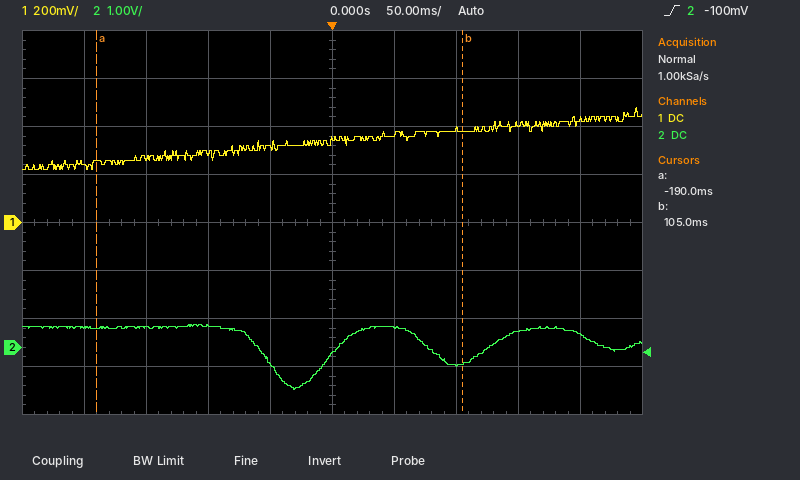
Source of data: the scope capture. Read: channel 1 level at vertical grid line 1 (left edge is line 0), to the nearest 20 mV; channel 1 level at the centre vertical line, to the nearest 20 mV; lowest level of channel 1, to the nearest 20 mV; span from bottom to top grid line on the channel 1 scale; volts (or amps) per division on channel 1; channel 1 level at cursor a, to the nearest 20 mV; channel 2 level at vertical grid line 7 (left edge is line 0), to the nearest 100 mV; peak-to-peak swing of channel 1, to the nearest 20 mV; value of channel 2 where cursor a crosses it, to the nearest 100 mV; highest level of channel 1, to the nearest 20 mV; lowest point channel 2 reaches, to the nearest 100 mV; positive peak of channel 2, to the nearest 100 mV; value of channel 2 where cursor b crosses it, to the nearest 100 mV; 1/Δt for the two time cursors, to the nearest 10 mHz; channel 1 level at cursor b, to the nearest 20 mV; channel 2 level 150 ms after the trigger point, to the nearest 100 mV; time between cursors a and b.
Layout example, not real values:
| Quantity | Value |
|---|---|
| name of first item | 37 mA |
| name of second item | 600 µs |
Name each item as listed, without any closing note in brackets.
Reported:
| Quantity | Value |
|---|---|
| channel 1 level at vertical grid line 1 (left edge is line 0), to the nearest 20 mV | 240 mV |
| channel 1 level at the centre vertical line, to the nearest 20 mV | 340 mV |
| lowest level of channel 1, to the nearest 20 mV | 220 mV |
| span from bottom to top grid line on the channel 1 scale | 1.6 V |
| volts (or amps) per division on channel 1 | 200 mV |
| channel 1 level at cursor a, to the nearest 20 mV | 260 mV |
| channel 2 level at vertical grid line 7 (left edge is line 0), to the nearest 100 mV | -400 mV |
| peak-to-peak swing of channel 1, to the nearest 20 mV | 260 mV |
| value of channel 2 where cursor a crosses it, to the nearest 100 mV | 400 mV |
| highest level of channel 1, to the nearest 20 mV | 480 mV |
| lowest point channel 2 reaches, to the nearest 100 mV | -900 mV |
| positive peak of channel 2, to the nearest 100 mV | 500 mV |
| value of channel 2 where cursor b crosses it, to the nearest 100 mV | -300 mV |
| 1/Δt for the two time cursors, to the nearest 10 mHz | 3.39 Hz |
| channel 1 level at cursor b, to the nearest 20 mV | 380 mV |
| channel 2 level 150 ms after the trigger point, to the nearest 100 mV | 300 mV |
| time between cursors a and b | 295 ms |
